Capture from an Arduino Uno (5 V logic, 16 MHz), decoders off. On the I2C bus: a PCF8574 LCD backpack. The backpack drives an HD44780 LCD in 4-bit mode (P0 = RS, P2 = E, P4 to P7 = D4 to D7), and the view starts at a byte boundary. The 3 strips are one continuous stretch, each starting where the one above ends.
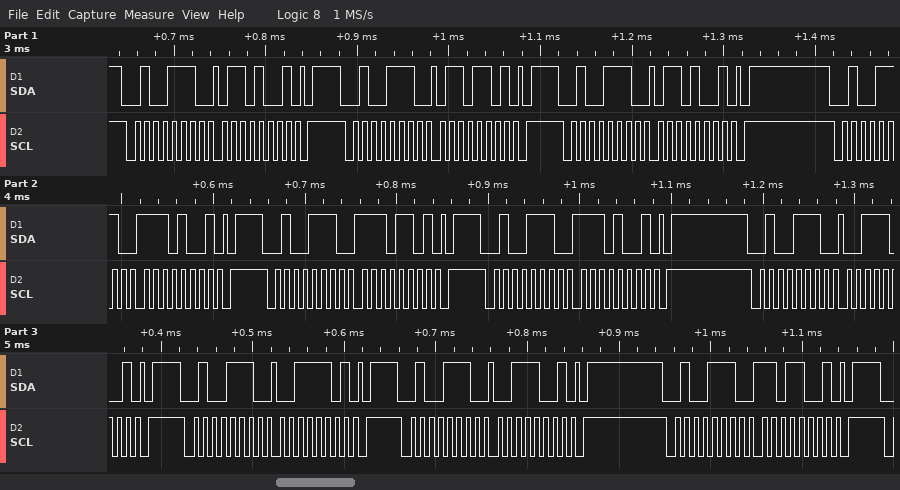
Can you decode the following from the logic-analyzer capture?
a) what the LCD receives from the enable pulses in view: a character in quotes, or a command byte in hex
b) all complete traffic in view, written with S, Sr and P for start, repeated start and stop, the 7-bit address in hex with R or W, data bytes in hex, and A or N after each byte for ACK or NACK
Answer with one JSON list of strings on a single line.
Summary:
["'n'", "S 27W A 69 A P S 27W A 6D A P S 27W A 69 A P S 27W A E9 A P S 27W A ED A P S 27W A E9 A P S 27W A 39 A P S 27W A 3D A P S 27W A 39 A P S 27W A D9 A P"]
